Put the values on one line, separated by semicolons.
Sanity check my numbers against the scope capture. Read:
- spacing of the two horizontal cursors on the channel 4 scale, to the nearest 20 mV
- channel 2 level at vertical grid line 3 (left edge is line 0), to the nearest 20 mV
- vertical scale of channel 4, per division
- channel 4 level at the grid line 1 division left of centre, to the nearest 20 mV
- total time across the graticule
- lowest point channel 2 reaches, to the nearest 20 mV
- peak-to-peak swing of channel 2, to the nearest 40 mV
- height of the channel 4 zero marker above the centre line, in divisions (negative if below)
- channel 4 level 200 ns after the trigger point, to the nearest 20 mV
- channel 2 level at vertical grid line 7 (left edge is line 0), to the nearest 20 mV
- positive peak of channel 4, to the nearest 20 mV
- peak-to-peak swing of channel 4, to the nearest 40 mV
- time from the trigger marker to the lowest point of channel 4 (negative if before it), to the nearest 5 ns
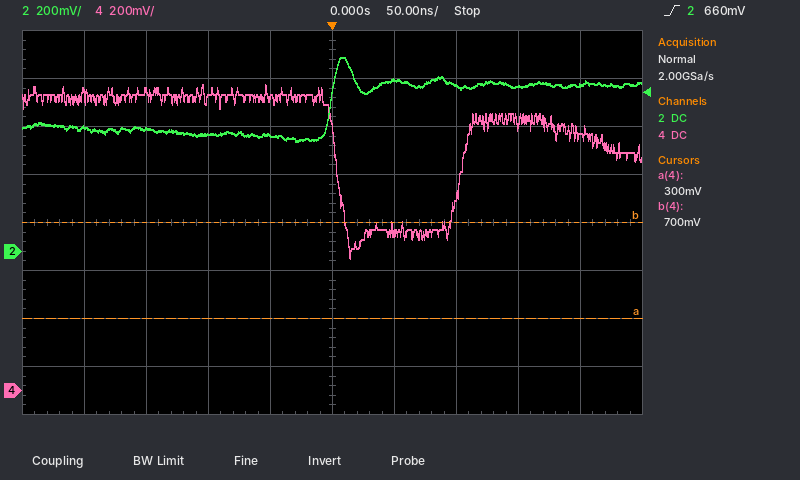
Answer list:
400 mV; 480 mV; 200 mV; 1.22 V; 500 ns; 460 mV; 360 mV; -3.5 div; 1.06 V; 700 mV; 1.28 V; 720 mV; +15 ns
